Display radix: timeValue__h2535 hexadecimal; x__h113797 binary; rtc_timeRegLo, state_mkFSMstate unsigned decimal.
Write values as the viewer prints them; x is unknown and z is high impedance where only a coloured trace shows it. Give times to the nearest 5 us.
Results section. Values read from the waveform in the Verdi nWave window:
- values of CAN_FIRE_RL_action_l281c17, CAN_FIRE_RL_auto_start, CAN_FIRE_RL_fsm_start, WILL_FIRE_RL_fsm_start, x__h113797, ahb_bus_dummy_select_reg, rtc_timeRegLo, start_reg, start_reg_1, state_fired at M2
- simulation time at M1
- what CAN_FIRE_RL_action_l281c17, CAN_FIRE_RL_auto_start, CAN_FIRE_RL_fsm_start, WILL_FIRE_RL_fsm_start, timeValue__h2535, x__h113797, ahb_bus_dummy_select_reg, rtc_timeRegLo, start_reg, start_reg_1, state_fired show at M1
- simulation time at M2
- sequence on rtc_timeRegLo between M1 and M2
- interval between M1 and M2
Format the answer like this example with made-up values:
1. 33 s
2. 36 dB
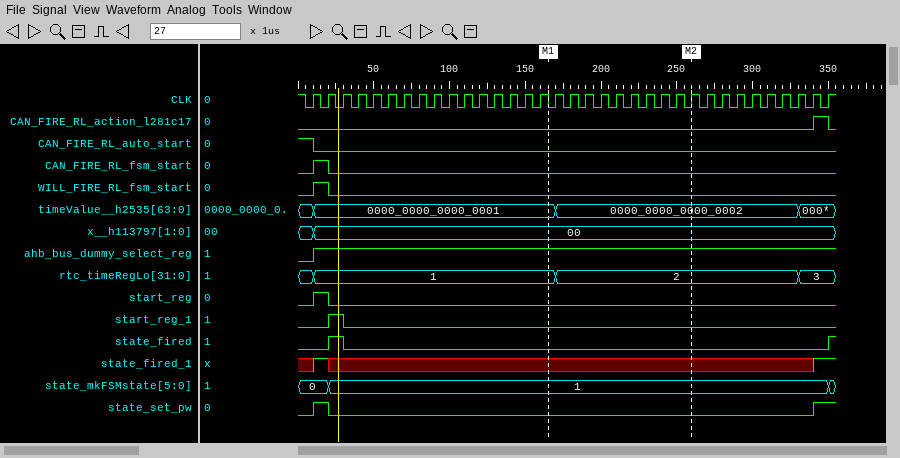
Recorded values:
1. CAN_FIRE_RL_action_l281c17=0, CAN_FIRE_RL_auto_start=0, CAN_FIRE_RL_fsm_start=0, WILL_FIRE_RL_fsm_start=0, x__h113797=00, ahb_bus_dummy_select_reg=1, rtc_timeRegLo=2, start_reg=0, start_reg_1=0, state_fired=0
2. 165 us
3. CAN_FIRE_RL_action_l281c17=0, CAN_FIRE_RL_auto_start=0, CAN_FIRE_RL_fsm_start=0, WILL_FIRE_RL_fsm_start=0, timeValue__h2535=0000_0000_0000_0001, x__h113797=00, ahb_bus_dummy_select_reg=1, rtc_timeRegLo=1, start_reg=0, start_reg_1=0, state_fired=0
4. 260 us
5. 1, 2
6. 95 us
